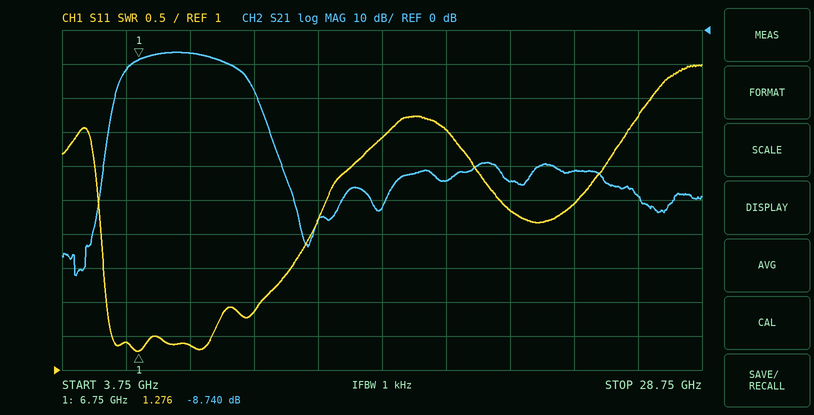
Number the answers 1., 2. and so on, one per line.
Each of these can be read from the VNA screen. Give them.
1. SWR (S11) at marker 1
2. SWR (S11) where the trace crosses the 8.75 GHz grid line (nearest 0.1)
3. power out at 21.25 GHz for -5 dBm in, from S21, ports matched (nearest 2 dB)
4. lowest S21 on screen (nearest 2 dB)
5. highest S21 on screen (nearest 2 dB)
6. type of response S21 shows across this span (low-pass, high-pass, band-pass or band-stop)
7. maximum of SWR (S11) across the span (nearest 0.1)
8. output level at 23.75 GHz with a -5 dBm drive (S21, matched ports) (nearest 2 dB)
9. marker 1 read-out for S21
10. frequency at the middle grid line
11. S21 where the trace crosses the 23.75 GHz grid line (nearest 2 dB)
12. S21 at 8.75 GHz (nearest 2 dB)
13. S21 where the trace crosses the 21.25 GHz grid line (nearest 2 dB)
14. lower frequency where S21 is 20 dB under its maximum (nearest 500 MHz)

1. 1.276
2. 1.4
3. -50 dBm
4. -72 dB
5. -6 dB
6. band-pass
7. 5.5
8. -46 dBm
9. -8.740 dB
10. 16.25 GHz
11. -42 dB
12. -6 dB
13. -44 dB
14. 5.5 GHz
